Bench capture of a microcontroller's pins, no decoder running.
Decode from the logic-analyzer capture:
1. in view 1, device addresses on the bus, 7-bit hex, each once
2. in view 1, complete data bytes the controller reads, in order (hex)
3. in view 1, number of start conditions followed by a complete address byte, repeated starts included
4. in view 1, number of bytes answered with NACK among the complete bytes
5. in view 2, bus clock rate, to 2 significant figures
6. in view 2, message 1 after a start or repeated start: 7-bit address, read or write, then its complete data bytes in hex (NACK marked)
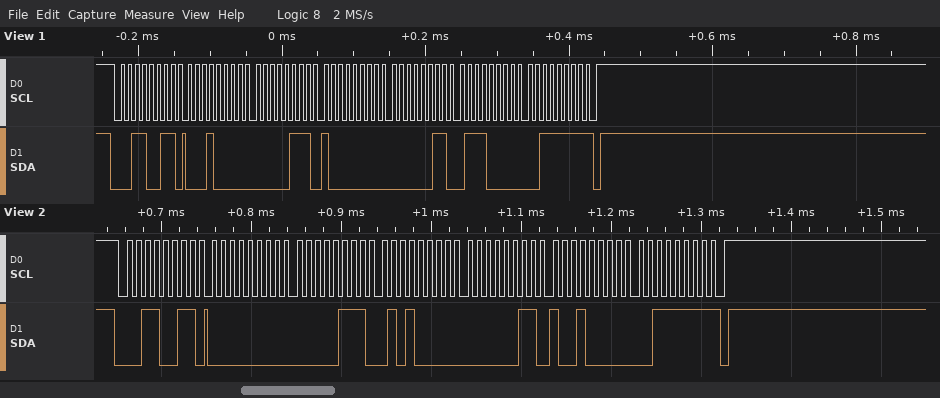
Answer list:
0x19
10 07 80 03 70 3F
1
1
100 kHz
0x19 read: 00 07 50 03 90 3F NACK
